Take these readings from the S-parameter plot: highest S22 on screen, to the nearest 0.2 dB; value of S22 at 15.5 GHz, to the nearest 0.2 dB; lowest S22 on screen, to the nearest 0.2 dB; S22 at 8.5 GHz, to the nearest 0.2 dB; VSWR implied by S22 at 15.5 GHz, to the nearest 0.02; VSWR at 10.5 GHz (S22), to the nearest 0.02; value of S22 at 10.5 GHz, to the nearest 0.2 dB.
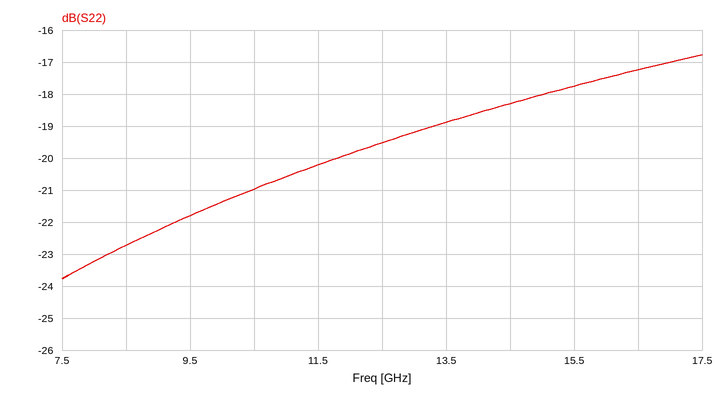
-16.8 dB
-17.8 dB
-23.8 dB
-22.8 dB
1.30
1.20
-21.0 dB
